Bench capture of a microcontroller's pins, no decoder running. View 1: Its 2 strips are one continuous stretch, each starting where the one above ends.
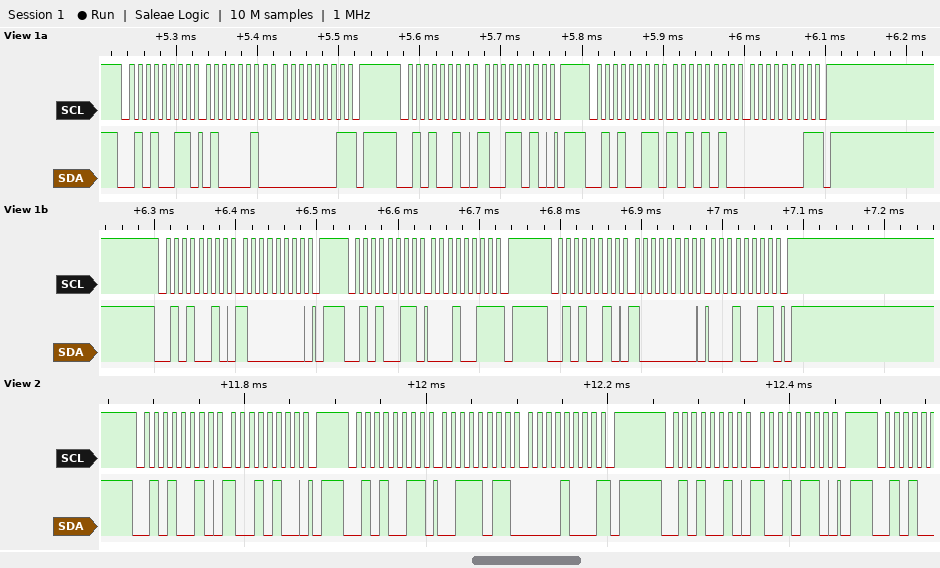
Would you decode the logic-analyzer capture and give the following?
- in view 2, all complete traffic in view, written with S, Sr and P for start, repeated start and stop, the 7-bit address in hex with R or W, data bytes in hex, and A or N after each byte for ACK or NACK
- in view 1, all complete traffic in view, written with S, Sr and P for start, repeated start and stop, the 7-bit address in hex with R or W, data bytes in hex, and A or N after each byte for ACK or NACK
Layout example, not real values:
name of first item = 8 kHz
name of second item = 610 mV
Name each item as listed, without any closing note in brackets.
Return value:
in view 2, all complete traffic in view, written with S, Sr and P for start, repeated start and stop, the 7-bit address in hex with R or W, data bytes in hex, and A or N after each byte for ACK or NACK = S 29W A 94 A P S 29R A 3B A 08 N P S 29W A 96 A P
in view 1, all complete traffic in view, written with S, Sr and P for start, repeated start and stop, the 7-bit address in hex with R or W, data bytes in hex, and A or N after each byte for ACK or NACK = S 29R A 42 A 01 N P S 29W A 9A A P S 29R A AA A 01 N P S 29W A 80 A P S 29R A 13 N P S 29W A 80 A 13 A P
